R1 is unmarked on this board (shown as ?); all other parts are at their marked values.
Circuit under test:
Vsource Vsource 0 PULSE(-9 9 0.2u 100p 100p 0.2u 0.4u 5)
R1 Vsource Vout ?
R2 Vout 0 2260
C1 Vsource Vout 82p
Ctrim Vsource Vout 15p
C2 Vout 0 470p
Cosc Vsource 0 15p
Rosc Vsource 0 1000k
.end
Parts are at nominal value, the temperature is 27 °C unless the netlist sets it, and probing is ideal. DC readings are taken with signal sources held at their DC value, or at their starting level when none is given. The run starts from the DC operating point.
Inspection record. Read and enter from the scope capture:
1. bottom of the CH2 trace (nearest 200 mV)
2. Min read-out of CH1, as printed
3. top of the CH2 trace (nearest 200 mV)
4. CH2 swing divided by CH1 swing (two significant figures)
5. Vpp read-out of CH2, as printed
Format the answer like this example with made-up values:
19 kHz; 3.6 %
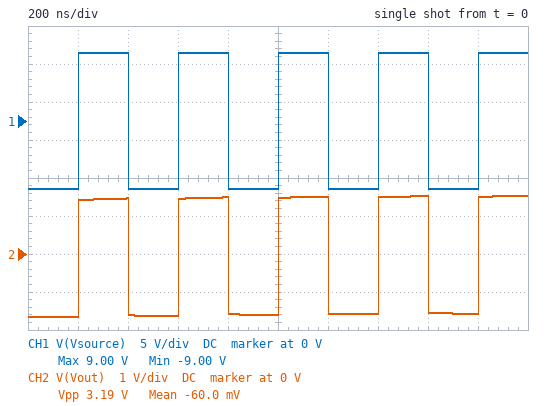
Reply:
-1.6 V; -9.00 V; 1.6 V; 0.18; 3.19 V
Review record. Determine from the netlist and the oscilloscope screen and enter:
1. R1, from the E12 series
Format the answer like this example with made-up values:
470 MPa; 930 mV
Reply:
10 kΩ
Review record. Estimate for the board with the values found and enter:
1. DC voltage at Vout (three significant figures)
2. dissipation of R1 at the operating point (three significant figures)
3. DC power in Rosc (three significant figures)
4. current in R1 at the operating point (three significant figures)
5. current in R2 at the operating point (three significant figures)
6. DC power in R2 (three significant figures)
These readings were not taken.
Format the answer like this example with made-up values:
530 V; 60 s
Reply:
-1.66 V; 5.39 mW; 81.0 µW; 734 µA; 734 µA; 1.22 mW
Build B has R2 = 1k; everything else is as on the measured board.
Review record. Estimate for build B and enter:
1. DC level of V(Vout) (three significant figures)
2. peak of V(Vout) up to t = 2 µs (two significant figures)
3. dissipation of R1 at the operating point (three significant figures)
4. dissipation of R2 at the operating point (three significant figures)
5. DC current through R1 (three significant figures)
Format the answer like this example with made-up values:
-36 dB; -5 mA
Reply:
-818 mV; 2.3 V; 6.69 mW; 669 µW; 818 µA
